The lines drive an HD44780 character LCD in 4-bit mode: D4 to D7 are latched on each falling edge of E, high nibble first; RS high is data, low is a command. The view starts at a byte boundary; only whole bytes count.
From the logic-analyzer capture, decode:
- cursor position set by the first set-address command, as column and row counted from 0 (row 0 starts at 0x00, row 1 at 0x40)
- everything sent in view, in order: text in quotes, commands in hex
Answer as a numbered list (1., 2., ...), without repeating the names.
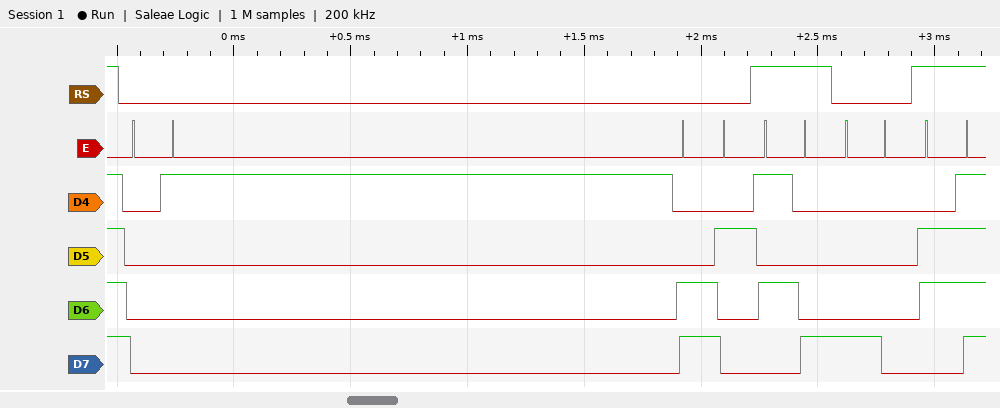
1. column 2, row 1
2. 0x01 0xC2 "X" 0x80 "o"
